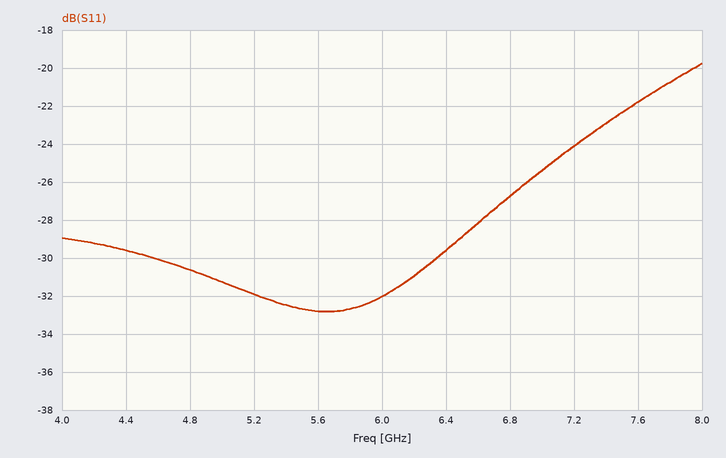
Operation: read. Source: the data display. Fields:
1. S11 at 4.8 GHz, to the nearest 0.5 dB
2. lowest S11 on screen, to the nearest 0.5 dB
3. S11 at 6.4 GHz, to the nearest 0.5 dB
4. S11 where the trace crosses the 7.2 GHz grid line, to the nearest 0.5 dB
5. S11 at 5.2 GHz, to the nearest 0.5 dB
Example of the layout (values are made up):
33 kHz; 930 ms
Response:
-30.5 dB; -33.0 dB; -29.5 dB; -24.0 dB; -32.0 dB
